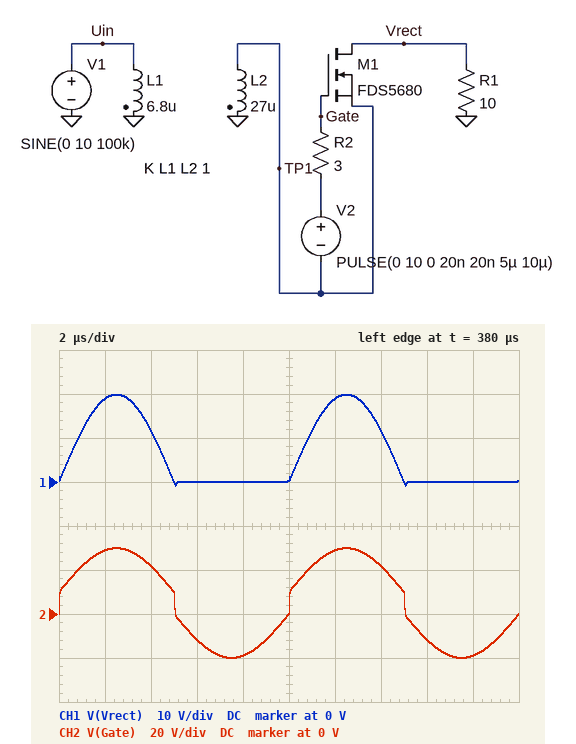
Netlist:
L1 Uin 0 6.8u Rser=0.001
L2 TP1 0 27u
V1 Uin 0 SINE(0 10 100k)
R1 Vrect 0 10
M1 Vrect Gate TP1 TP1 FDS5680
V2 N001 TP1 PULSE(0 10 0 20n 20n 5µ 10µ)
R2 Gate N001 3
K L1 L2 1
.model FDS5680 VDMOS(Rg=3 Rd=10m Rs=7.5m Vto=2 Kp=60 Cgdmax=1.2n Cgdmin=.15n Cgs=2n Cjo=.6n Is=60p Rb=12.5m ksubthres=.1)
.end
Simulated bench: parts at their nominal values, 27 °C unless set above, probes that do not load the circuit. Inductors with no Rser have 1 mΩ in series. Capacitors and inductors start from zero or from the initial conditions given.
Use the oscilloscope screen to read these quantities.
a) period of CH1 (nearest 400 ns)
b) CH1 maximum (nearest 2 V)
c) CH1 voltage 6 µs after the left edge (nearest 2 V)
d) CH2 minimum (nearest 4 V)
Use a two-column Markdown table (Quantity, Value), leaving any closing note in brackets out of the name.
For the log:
| Quantity | Value |
|---|---|
| period of CH1 | 10.0 µs |
| CH1 maximum | 20 V |
| CH1 voltage 6 µs after the left edge | 0 V |
| CH2 minimum | -20 V |
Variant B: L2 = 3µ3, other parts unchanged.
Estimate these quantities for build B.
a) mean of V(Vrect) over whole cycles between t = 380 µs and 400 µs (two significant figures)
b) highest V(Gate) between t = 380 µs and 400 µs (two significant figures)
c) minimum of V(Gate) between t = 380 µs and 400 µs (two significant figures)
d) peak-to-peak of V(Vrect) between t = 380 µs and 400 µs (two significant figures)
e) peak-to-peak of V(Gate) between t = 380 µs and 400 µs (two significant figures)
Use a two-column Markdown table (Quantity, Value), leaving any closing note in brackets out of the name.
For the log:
| Quantity | Value |
|---|---|
| mean of V(Vrect) over whole cycles between t = 380 µs and 400 µs | 2.2 V |
| highest V(Gate) between t = 380 µs and 400 µs | 17 V |
| minimum of V(Gate) between t = 380 µs and 400 µs | -7.0 V |
| peak-to-peak of V(Vrect) between t = 380 µs and 400 µs | 7.6 V |
| peak-to-peak of V(Gate) between t = 380 µs and 400 µs | 24 V |
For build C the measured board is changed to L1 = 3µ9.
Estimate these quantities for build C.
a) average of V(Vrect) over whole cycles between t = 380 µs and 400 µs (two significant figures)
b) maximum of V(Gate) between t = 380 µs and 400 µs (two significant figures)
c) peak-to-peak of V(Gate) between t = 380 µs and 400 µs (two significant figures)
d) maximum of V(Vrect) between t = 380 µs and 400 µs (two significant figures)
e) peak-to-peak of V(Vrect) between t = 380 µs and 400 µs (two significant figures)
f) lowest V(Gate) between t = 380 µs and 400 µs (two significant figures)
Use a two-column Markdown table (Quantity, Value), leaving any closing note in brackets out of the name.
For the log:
| Quantity | Value |
|---|---|
| average of V(Vrect) over whole cycles between t = 380 µs and 400 µs | 8.3 V |
| maximum of V(Gate) between t = 380 µs and 400 µs | 36 V |
| peak-to-peak of V(Gate) between t = 380 µs and 400 µs | 63 V |
| maximum of V(Vrect) between t = 380 µs and 400 µs | 26 V |
| peak-to-peak of V(Vrect) between t = 380 µs and 400 µs | 27 V |
| lowest V(Gate) between t = 380 µs and 400 µs | -26 V |
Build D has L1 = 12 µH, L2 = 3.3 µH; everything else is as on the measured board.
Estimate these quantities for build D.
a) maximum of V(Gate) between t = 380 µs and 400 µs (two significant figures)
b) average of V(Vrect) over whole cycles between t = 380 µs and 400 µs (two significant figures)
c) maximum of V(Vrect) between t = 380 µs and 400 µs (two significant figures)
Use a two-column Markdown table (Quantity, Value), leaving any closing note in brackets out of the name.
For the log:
| Quantity | Value |
|---|---|
| maximum of V(Gate) between t = 380 µs and 400 µs | 15 V |
| average of V(Vrect) over whole cycles between t = 380 µs and 400 µs | 1.7 V |
| maximum of V(Vrect) between t = 380 µs and 400 µs | 5.2 V |
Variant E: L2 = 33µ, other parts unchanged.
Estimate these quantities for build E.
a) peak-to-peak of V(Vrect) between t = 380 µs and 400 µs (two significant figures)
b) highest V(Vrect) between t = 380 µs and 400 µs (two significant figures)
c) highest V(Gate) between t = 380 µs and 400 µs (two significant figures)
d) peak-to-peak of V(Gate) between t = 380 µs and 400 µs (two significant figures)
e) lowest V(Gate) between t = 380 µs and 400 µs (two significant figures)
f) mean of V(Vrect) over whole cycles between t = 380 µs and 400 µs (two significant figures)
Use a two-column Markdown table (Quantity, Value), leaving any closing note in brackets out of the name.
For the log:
| Quantity | Value |
|---|---|
| peak-to-peak of V(Vrect) between t = 380 µs and 400 µs | 23 V |
| highest V(Vrect) between t = 380 µs and 400 µs | 22 V |
| highest V(Gate) between t = 380 µs and 400 µs | 32 V |
| peak-to-peak of V(Gate) between t = 380 µs and 400 µs | 54 V |
| lowest V(Gate) between t = 380 µs and 400 µs | -22 V |
| mean of V(Vrect) over whole cycles between t = 380 µs and 400 µs | 7.0 V |
